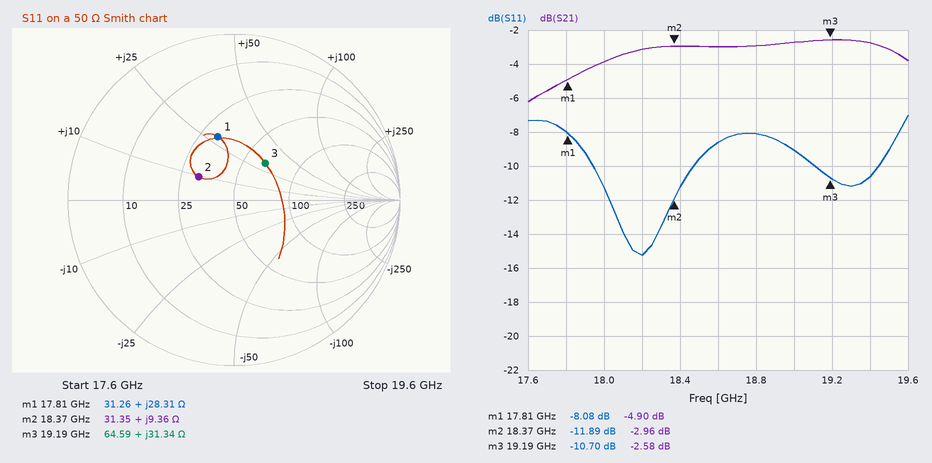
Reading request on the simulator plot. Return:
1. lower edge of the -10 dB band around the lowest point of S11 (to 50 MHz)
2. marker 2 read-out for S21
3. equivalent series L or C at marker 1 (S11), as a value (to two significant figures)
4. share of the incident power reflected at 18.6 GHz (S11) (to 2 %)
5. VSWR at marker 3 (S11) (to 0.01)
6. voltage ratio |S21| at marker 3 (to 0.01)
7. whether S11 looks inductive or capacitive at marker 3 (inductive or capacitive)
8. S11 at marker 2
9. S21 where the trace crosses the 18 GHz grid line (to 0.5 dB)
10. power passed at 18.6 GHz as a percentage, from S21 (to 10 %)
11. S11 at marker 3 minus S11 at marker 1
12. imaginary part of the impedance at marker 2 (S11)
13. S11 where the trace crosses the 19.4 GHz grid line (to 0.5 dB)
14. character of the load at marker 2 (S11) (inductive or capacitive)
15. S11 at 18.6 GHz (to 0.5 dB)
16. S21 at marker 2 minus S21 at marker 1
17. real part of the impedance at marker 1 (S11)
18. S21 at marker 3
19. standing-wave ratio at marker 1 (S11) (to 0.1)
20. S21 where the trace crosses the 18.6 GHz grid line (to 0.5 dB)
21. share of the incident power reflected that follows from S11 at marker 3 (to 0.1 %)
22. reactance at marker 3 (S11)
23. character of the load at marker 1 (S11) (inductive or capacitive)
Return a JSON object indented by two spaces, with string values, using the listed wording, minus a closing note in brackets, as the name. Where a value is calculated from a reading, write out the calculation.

{
  "lower edge of the -10 dB band around the lowest point of S11": "17.95 GHz",
  "marker 2 read-out for S21": "-2.96 dB",
  "equivalent series L or C at marker 1 (S11), as a value": "L = 28.31 Ω/(2π × 17.81 GHz) ≈ 253 pH, so 250 pH to two significant figures",
  "share of the incident power reflected at 18.6 GHz (S11)": "10^(-8.5/10) ≈ 14 %",
  "VSWR at marker 3 (S11)": "1.82",
  "voltage ratio |S21| at marker 3": "10^(-2.58/20) ≈ 0.74",
  "whether S11 looks inductive or capacitive at marker 3": "inductive",
  "S11 at marker 2": "-11.89 dB",
  "S21 where the trace crosses the 18 GHz grid line": "-4.0 dB",
  "power passed at 18.6 GHz as a percentage, from S21": "10^(-3/10) ≈ 50 %",
  "S11 at marker 3 minus S11 at marker 1": "-10.7 − (-8.08) = -2.62 dB",
  "imaginary part of the impedance at marker 2": "+9.36 Ω",
  "S11 where the trace crosses the 19.4 GHz grid line": "-10.5 dB",
  "character of the load at marker 2 (S11)": "inductive",
  "S11 at 18.6 GHz": "-8.5 dB",
  "S21 at marker 2 minus S21 at marker 1": "-2.96 − (-4.9) = 1.94 dB",
  "real part of the impedance at marker 1": "31.26 Ω",
  "S21 at marker 3": "-2.58 dB",
  "standing-wave ratio at marker 1 (S11)": "2.3",
  "S21 where the trace crosses the 18.6 GHz grid line": "-3.0 dB",
  "share of the incident power reflected that follows from S11 at marker 3": "10^(-10.7/10) ≈ 8.5 %",
  "reactance at marker 3": "+31.34 Ω",
  "character of the load at marker 1 (S11)": "inductive"
}
